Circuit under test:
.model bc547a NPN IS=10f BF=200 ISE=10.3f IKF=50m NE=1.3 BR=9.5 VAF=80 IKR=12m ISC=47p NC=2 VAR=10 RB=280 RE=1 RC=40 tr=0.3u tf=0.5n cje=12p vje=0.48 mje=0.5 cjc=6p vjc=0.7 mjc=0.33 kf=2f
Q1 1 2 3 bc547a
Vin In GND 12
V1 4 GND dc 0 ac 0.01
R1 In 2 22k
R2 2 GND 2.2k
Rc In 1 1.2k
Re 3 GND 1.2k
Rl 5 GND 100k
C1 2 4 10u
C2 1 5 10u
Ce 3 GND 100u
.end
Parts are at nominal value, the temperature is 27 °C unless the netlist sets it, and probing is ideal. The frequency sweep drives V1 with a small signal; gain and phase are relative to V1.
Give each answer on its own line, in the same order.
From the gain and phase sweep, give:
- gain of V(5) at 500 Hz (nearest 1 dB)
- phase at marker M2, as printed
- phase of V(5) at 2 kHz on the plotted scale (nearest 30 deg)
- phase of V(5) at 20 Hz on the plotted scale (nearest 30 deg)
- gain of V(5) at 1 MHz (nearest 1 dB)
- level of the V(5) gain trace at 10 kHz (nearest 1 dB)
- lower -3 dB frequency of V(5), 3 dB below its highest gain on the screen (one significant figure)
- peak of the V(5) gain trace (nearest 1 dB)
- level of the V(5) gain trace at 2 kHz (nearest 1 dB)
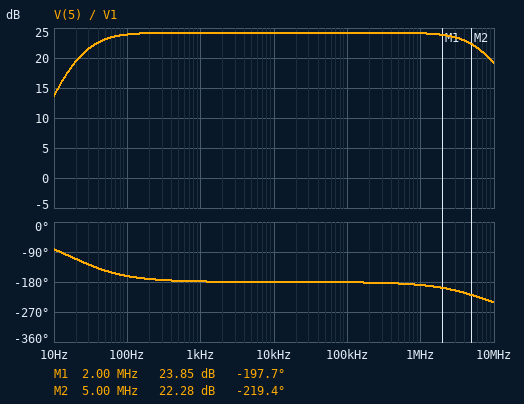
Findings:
24 dB
-219.4 deg
-180 deg
-120 deg
24 dB
24 dB
30 Hz
24 dB
24 dB
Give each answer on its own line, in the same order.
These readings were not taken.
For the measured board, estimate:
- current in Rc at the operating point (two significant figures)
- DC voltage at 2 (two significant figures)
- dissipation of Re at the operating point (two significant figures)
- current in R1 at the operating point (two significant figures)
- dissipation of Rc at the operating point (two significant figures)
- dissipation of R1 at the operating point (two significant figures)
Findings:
380 µA
1.1 V
170 µW
500 µA
170 µW
5.4 mW
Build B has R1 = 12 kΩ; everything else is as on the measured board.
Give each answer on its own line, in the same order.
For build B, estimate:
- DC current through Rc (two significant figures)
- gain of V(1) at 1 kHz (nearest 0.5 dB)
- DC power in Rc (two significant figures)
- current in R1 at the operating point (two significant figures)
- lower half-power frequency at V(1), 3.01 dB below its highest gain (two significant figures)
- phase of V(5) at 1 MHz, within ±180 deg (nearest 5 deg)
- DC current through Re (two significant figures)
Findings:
980 µA
32.0 dB
1.2 mW
850 µA
60 Hz
165 deg
990 µA
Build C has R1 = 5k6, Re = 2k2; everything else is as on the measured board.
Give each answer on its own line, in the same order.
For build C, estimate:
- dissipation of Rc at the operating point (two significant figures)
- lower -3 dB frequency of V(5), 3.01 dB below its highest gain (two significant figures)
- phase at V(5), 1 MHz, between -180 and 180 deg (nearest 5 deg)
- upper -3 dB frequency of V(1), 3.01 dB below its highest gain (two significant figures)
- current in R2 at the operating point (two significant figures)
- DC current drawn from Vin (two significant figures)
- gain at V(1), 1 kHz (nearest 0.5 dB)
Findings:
1.8 mW
71 Hz
160 deg
3.0 MHz
1.5 mA
2.8 mA
33.5 dB
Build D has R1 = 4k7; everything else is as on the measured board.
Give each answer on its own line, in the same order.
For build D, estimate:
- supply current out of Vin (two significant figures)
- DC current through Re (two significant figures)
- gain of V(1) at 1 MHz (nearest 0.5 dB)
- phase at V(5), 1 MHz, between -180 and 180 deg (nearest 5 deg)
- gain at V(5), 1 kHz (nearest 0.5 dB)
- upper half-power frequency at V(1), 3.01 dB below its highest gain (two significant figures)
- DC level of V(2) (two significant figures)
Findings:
4.3 mA
2.6 mA
37.0 dB
150 deg
38.5 dB
1.7 MHz
3.8 V
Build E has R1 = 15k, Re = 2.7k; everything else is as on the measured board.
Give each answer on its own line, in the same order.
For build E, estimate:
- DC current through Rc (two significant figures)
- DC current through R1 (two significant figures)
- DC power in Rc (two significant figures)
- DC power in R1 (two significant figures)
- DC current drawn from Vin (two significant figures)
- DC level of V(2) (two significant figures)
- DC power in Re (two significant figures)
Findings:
330 µA
700 µA
130 µW
7.3 mW
1.0 mA
1.5 V
300 µW
